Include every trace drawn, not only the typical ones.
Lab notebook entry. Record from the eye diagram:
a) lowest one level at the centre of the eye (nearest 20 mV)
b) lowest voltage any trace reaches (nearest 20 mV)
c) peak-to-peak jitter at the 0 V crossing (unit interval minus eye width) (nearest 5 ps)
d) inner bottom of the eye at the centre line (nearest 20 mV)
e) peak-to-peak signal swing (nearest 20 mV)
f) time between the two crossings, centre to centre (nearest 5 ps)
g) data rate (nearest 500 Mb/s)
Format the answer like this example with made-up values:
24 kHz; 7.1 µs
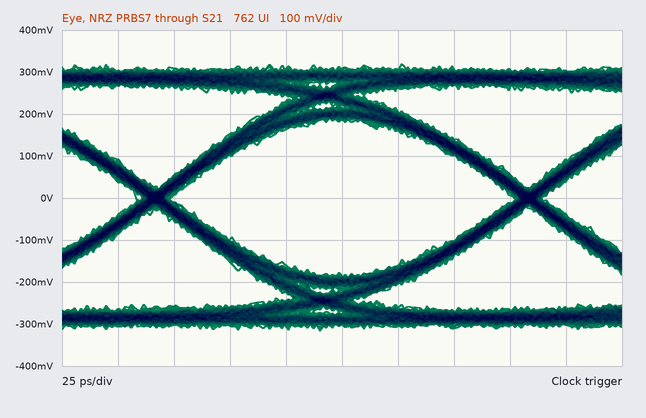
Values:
180 mV; -320 mV; 15 ps; -180 mV; 640 mV; 165 ps; 6.0 Gb/s
